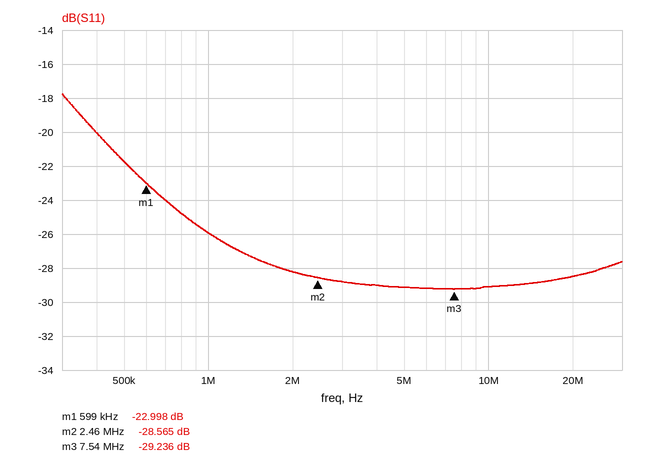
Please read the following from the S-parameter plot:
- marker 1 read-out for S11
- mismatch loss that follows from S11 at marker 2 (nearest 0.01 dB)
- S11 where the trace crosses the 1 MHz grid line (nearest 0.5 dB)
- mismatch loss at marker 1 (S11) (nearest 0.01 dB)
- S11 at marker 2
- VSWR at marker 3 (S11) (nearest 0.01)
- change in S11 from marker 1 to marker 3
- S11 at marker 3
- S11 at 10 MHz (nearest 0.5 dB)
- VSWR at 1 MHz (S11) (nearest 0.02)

-22.998 dB
0.01 dB
-26.0 dB
0.02 dB
-28.565 dB
1.07
-6.238 dB
-29.236 dB
-29.0 dB
1.10
